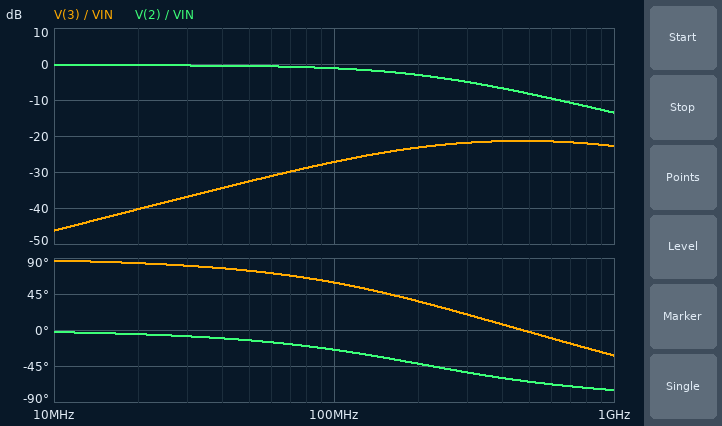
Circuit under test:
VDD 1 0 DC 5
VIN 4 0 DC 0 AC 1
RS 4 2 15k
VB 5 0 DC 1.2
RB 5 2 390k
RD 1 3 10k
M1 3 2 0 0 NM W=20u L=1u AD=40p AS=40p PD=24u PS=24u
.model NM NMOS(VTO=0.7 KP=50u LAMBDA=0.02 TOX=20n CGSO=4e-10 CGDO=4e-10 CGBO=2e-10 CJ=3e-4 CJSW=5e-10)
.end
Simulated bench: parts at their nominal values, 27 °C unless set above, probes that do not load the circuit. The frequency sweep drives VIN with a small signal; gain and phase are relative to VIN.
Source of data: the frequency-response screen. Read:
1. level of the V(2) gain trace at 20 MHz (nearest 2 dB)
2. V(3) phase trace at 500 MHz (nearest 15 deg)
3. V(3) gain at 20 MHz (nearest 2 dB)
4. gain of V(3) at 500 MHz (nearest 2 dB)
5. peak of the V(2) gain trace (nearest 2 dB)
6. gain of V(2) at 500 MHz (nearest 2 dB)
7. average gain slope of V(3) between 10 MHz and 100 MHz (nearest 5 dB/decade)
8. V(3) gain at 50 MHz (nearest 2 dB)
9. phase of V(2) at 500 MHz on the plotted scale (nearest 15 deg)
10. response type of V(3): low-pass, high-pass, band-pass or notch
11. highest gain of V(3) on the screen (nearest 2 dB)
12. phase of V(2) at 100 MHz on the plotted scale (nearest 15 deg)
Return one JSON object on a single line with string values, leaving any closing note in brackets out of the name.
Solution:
{"level of the V(2) gain trace at 20 MHz": "0 dB", "V(3) phase trace at 500 MHz": "0 deg", "V(3) gain at 20 MHz": "-40 dB", "gain of V(3) at 500 MHz": "-22 dB", "peak of the V(2) gain trace": "0 dB", "gain of V(2) at 500 MHz": "-8 dB", "average gain slope of V(3) between 10 MHz and 100 MHz": "20 dB/decade", "V(3) gain at 50 MHz": "-32 dB", "phase of V(2) at 500 MHz on the plotted scale": "-60 deg", "response type of V(3): low-pass, high-pass, band-pass or notch": "high-pass", "highest gain of V(3) on the screen": "-22 dB", "phase of V(2) at 100 MHz on the plotted scale": "-30 deg"}
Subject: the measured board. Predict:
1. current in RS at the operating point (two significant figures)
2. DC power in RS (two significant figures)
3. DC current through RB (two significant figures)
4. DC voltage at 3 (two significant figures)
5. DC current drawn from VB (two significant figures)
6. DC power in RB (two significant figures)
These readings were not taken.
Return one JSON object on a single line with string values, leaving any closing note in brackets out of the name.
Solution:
{"current in RS at the operating point": "3.0 µA", "DC power in RS": "130 nW", "DC current through RB": "3.0 µA", "DC voltage at 3": "5.0 V", "DC current drawn from VB": "3.0 µA", "DC power in RB": "3.4 µW"}
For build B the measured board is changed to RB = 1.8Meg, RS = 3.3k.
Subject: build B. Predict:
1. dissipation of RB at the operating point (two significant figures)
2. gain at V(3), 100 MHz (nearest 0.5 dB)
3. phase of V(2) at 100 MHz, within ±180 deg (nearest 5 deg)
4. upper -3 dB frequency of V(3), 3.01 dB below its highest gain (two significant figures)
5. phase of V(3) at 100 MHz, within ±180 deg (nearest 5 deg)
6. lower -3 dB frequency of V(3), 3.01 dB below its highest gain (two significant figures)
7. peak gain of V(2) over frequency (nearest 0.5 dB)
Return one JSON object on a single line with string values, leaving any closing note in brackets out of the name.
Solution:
{"dissipation of RB at the operating point": "800 nW", "gain at V(3), 100 MHz": "-26.0 dB", "phase of V(2) at 100 MHz, within ±180 deg": "-5 deg", "upper -3 dB frequency of V(3), 3.01 dB below its highest gain": "2.4 GHz", "phase of V(3) at 100 MHz, within ±180 deg": "80 deg", "lower -3 dB frequency of V(3), 3.01 dB below its highest gain": "400 MHz", "peak gain of V(2) over frequency": "0 dB"}
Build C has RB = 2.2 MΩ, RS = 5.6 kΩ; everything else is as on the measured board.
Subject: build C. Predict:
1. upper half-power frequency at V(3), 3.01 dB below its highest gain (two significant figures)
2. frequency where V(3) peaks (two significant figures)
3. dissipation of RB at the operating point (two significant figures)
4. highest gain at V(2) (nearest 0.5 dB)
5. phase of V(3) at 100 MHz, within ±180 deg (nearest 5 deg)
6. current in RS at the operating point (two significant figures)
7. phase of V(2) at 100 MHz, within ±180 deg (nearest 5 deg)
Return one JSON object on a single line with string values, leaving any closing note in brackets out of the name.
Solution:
{"upper half-power frequency at V(3), 3.01 dB below its highest gain": "1.9 GHz", "frequency where V(3) peaks": "760 MHz", "dissipation of RB at the operating point": "650 nW", "highest gain at V(2)": "0 dB", "phase of V(3) at 100 MHz, within ±180 deg": "75 deg", "current in RS at the operating point": "540 nA", "phase of V(2) at 100 MHz, within ±180 deg": "-10 deg"}
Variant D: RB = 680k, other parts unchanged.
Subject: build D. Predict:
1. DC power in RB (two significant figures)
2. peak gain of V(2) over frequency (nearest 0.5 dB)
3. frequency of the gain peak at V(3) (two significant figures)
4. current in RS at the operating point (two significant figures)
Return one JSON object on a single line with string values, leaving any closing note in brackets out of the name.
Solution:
{"DC power in RB": "2.0 µW", "peak gain of V(2) over frequency": "0 dB", "frequency of the gain peak at V(3)": "470 MHz", "current in RS at the operating point": "1.7 µA"}
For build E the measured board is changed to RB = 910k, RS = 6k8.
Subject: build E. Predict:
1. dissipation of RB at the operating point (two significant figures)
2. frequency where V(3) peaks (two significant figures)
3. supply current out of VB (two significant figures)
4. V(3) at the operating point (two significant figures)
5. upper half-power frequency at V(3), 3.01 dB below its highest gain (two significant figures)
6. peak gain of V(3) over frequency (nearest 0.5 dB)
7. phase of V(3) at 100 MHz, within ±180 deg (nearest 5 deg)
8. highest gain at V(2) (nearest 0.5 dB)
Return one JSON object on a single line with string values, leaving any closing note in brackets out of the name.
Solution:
{"dissipation of RB at the operating point": "1.6 µW", "frequency where V(3) peaks": "690 MHz", "supply current out of VB": "1.3 µA", "V(3) at the operating point": "5.0 V", "upper half-power frequency at V(3), 3.01 dB below its highest gain": "1.8 GHz", "peak gain of V(3) over frequency": "-16.0 dB", "phase of V(3) at 100 MHz, within ±180 deg": "70 deg", "highest gain at V(2)": "0 dB"}
